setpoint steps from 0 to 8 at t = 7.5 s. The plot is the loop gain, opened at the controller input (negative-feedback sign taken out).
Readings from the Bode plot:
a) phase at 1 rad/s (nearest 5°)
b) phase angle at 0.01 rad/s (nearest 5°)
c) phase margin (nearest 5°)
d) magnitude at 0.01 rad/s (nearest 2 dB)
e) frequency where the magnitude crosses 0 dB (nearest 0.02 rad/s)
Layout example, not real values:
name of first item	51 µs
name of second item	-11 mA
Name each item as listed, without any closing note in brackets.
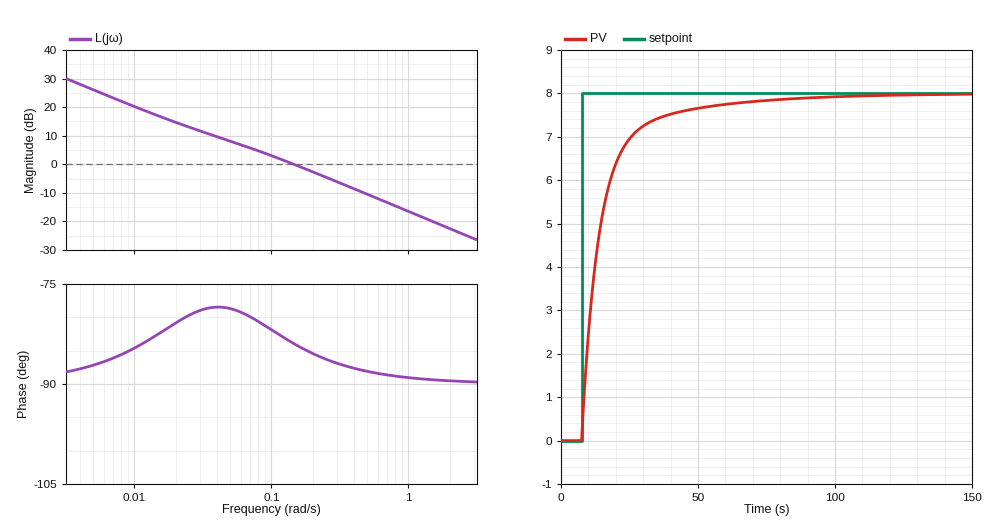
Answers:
phase at 1 rad/s	-90°
phase angle at 0.01 rad/s	-85°
phase margin	95°
magnitude at 0.01 rad/s	20 dB
frequency where the magnitude crosses 0 dB	0.14 rad/s
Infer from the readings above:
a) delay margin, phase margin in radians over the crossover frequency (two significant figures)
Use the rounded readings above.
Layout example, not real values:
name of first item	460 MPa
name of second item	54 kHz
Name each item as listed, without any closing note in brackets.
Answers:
delay margin, phase margin in radians over the crossover frequency	12 s
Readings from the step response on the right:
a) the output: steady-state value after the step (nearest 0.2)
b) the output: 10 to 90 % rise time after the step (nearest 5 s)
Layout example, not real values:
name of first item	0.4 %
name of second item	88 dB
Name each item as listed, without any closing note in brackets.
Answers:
the output: steady-state value after the step	8.0
the output: 10 to 90 % rise time after the step	20 s
